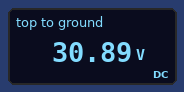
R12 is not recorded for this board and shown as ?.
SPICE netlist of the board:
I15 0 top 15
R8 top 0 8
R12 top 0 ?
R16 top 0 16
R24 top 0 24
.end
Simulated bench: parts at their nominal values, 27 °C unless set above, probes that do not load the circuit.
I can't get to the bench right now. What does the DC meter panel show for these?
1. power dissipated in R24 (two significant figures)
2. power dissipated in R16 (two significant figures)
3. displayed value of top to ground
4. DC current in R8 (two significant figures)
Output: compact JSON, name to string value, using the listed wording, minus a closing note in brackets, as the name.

{"power dissipated in R24": "40 W", "power dissipated in R16": "60 W", "displayed value of top to ground": "30.89 V", "DC current in R8": "3.9 A"}
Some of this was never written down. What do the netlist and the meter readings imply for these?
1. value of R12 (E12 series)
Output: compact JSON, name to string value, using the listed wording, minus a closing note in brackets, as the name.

{"value of R12": "3.9 Ω"}
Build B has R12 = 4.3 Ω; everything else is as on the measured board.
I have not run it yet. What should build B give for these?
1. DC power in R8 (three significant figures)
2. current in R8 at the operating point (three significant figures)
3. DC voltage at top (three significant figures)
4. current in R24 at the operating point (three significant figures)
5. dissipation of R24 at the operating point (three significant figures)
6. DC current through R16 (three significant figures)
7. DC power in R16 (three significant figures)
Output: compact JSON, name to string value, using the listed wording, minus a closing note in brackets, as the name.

{"DC power in R8": "132 W", "current in R8 at the operating point": "4.06 A", "DC voltage at top": "32.5 V", "current in R24 at the operating point": "1.35 A", "dissipation of R24 at the operating point": "44.0 W", "DC current through R16": "2.03 A", "DC power in R16": "66.0 W"}
